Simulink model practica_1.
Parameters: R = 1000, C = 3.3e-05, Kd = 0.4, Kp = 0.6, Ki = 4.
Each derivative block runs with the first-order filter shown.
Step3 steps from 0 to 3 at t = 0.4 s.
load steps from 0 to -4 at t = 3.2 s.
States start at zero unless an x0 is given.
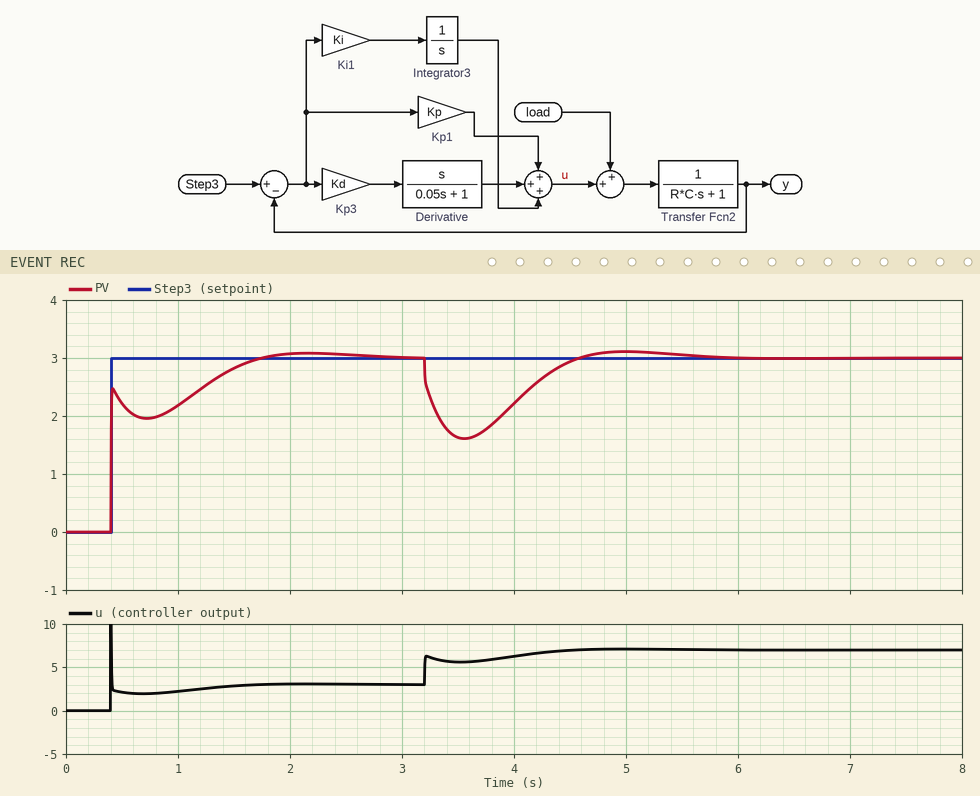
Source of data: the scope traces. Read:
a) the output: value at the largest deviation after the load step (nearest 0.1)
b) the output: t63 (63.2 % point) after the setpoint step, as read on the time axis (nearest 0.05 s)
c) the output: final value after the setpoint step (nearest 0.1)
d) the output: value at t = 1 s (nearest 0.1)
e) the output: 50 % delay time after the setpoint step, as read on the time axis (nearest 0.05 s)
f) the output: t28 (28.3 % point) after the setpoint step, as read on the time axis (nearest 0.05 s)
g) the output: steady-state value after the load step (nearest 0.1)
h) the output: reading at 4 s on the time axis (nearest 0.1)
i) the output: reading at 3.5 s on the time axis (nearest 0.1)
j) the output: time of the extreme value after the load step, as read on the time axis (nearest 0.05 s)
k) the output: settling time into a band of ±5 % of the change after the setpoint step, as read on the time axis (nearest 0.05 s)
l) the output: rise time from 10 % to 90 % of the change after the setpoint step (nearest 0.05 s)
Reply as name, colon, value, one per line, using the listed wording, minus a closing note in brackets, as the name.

the output: value at the largest deviation after the load step: 1.6
the output: t63 (63.2 % point) after the setpoint step, as read on the time axis: 0.40 s
the output: final value after the setpoint step: 3.0
the output: value at t = 1 s: 2.2
the output: 50 % delay time after the setpoint step, as read on the time axis: 0.40 s
the output: t28 (28.3 % point) after the setpoint step, as read on the time axis: 0.40 s
the output: steady-state value after the load step: 3.0
the output: reading at 4 s on the time axis: 2.2
the output: reading at 3.5 s on the time axis: 1.6
the output: time of the extreme value after the load step, as read on the time axis: 3.55 s
the output: settling time into a band of ±5 % of the change after the setpoint step, as read on the time axis: 1.55 s
the output: rise time from 10 % to 90 % of the change after the setpoint step: 1.00 s
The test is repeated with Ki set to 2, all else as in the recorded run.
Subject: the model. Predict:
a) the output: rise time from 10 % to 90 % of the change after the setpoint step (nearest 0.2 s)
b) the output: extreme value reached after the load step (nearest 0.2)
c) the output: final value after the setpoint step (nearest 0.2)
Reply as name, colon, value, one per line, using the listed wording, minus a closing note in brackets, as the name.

the output: rise time from 10 % to 90 % of the change after the setpoint step: 1.6 s
the output: extreme value reached after the load step: 1.4
the output: final value after the setpoint step: 3.0
